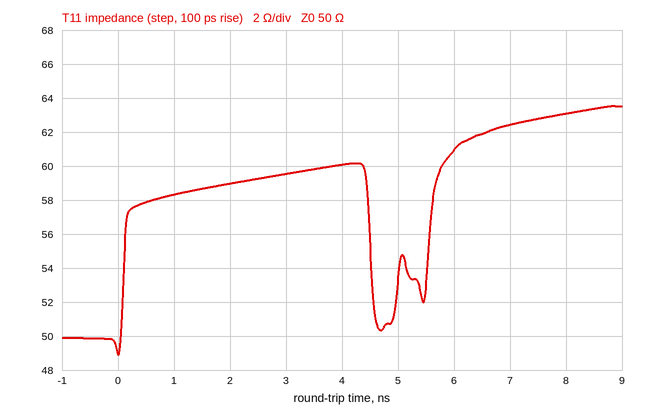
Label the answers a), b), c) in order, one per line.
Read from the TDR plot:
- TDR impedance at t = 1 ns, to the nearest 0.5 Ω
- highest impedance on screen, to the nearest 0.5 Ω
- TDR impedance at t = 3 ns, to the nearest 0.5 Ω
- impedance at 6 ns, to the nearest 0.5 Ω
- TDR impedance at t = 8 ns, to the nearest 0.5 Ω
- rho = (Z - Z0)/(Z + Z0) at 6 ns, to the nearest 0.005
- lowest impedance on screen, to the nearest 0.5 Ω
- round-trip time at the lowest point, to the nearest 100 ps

a) 58.5 Ω
b) 63.5 Ω
c) 59.5 Ω
d) 61.0 Ω
e) 63.0 Ω
f) +0.100
g) 49.0 Ω
h) 0.0 ns
